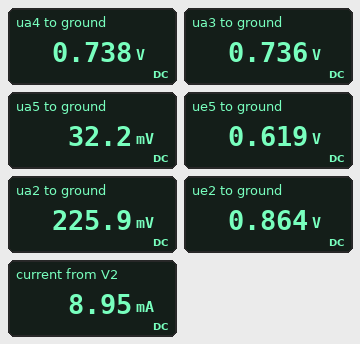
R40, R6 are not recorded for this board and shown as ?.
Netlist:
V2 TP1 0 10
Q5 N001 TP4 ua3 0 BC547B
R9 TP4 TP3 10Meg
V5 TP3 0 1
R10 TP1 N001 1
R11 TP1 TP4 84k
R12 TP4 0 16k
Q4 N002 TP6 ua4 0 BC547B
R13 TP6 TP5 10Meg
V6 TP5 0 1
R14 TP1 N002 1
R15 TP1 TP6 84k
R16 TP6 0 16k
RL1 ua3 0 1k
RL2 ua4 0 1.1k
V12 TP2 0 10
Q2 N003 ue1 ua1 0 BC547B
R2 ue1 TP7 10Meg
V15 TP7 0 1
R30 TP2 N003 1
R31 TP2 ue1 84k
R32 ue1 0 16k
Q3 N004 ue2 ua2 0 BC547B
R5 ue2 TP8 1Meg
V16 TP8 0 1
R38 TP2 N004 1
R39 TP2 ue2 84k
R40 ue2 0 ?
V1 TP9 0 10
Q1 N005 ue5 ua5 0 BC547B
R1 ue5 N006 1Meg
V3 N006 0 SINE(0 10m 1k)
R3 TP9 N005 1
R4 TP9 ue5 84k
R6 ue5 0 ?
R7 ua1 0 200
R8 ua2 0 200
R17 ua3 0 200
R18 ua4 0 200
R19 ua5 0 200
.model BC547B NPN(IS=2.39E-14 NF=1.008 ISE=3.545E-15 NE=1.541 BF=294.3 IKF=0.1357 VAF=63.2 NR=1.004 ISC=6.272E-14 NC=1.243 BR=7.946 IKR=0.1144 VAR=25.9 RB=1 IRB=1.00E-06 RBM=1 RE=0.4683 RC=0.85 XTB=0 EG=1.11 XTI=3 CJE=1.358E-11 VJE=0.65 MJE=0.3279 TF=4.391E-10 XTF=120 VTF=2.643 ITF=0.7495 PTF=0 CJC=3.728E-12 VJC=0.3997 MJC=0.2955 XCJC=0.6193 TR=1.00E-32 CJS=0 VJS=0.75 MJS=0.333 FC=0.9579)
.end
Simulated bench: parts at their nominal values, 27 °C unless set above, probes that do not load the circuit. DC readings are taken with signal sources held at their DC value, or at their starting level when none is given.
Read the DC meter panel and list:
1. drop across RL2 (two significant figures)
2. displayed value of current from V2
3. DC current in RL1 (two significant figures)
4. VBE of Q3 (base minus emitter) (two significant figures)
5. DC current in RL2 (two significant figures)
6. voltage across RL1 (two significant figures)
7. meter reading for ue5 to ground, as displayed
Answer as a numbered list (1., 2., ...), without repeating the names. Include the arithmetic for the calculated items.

1. 738 mV = 740 mV
2. 8.95 mA
3. (736 mV) / 1 kΩ = 740 µA
4. 864 mV - 225.9 mV = 640 mV
5. (738 mV) / 1.1 kΩ = 670 µA
6. 736 mV = 740 mV
7. 0.619 V
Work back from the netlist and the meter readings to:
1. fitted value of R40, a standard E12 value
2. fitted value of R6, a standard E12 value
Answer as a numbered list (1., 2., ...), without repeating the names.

1. 8.2 kΩ
2. 5.6 kΩ
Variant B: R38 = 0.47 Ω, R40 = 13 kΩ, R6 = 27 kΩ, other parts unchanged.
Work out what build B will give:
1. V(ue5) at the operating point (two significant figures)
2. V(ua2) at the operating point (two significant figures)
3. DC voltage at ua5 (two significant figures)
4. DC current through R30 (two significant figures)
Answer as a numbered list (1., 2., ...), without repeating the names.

1. 2.0 V
2. 570 mV
3. 1.3 V
4. 3.8 mA
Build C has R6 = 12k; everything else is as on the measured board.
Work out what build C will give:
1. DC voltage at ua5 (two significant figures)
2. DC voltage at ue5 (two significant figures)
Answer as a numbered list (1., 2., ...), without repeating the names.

1. 500 mV
2. 1.2 V
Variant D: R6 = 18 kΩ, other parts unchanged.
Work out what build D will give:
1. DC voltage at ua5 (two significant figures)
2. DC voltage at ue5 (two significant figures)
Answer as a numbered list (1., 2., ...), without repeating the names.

1. 860 mV
2. 1.5 V
